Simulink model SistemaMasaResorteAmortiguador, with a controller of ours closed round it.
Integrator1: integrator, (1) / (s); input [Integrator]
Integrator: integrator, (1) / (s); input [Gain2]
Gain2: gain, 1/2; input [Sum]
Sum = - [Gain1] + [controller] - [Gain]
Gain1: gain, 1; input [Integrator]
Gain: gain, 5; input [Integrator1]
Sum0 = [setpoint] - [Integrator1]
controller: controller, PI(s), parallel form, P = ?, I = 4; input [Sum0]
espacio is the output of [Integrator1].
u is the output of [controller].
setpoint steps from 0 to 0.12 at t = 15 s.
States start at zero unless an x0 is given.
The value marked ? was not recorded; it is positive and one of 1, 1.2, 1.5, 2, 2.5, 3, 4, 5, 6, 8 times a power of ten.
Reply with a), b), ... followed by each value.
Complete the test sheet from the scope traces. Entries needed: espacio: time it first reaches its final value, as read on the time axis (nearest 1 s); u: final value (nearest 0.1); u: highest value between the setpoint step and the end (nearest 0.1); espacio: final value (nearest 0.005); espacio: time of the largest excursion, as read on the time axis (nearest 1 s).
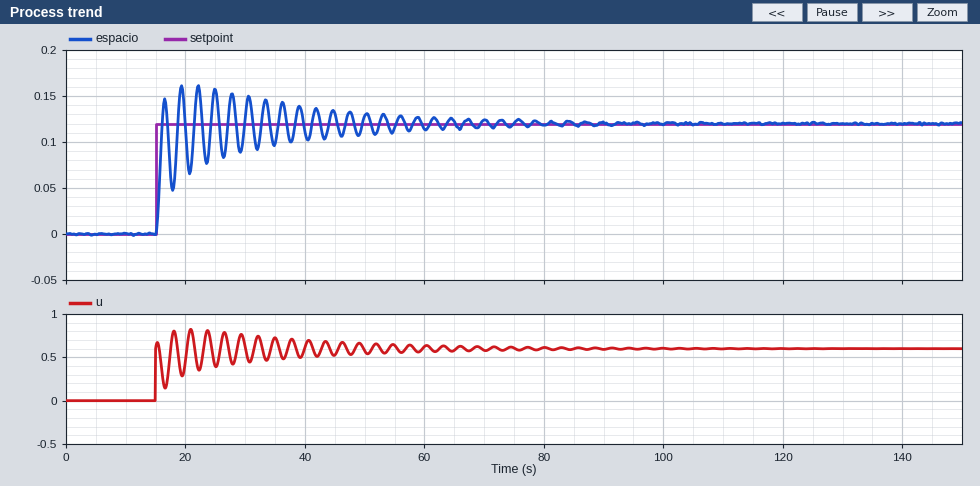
a) 16 s
b) 0.6
c) 0.8
d) 0.120
e) 22 s
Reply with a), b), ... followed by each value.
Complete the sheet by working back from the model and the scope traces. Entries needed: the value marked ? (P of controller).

a) 5
